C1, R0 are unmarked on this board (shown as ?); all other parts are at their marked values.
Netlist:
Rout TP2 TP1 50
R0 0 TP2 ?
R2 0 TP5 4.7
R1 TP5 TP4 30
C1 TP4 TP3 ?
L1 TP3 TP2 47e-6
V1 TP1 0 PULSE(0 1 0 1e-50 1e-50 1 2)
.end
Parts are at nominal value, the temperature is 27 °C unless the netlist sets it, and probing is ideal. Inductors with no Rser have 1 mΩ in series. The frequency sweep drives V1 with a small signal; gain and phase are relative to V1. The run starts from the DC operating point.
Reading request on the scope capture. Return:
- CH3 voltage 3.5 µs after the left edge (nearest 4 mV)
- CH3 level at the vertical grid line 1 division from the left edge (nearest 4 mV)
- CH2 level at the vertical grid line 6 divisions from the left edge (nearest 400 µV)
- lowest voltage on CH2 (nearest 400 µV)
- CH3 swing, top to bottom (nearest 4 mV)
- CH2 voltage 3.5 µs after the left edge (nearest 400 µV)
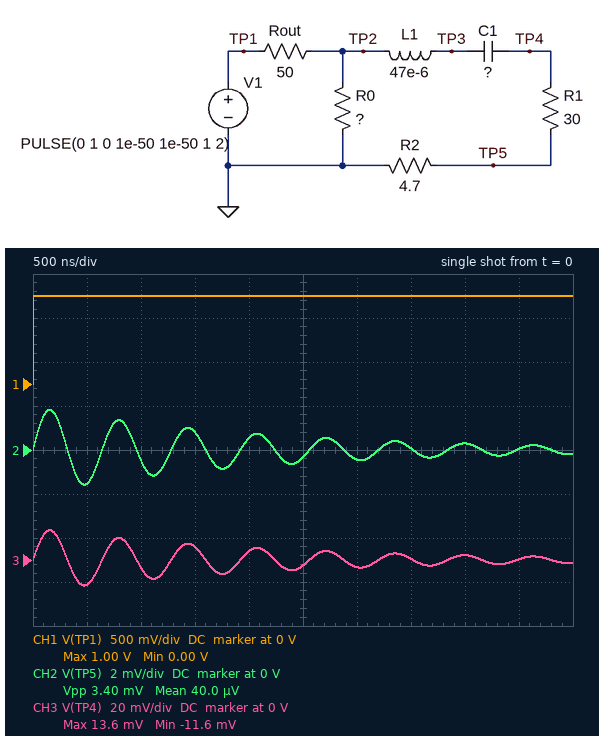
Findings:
0 V
-12 mV
-400 µV
-1.6 mV
24 mV
0 V
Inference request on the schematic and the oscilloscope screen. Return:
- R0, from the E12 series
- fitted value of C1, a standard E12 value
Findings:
12 Ω
220 pF
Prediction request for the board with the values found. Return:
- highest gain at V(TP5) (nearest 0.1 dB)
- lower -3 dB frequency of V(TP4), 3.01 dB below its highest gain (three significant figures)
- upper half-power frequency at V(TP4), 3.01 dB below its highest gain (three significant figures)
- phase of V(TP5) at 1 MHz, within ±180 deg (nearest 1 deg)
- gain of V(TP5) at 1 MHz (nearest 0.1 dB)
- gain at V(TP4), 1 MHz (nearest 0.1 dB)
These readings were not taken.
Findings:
-33.8 dB
1.49 MHz
1.64 MHz
84 deg
-53.5 dB
-36.1 dB
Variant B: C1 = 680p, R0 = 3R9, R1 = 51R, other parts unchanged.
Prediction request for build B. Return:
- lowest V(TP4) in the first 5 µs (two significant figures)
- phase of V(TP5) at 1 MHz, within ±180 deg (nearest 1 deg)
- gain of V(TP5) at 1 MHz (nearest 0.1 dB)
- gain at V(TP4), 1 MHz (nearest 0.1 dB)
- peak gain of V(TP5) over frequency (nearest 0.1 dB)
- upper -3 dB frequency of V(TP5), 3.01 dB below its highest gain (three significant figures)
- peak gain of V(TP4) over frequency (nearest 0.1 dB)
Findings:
-9.1 mV
-46 deg
-48.0 dB
-26.5 dB
-44.8 dB
996 kHz
-23.4 dB
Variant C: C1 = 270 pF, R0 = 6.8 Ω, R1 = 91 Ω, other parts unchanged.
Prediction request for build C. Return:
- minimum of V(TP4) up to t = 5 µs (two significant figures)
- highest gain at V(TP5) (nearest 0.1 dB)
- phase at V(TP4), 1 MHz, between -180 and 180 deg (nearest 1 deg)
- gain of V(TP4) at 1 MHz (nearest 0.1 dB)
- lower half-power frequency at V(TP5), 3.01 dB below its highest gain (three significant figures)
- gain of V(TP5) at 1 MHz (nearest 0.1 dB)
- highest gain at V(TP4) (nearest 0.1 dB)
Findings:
-16 mV
-45.1 dB
71 deg
-28.7 dB
1.25 MHz
-54.9 dB
-19.0 dB
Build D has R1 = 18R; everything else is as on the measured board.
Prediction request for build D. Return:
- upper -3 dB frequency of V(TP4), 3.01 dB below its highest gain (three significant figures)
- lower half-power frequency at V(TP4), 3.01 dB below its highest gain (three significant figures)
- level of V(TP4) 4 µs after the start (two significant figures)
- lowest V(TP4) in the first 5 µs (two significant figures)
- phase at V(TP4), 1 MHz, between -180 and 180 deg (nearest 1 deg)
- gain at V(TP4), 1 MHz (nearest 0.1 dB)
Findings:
1.62 MHz
1.51 MHz
2.4 mV
-8.1 mV
86 deg
-39.8 dB
